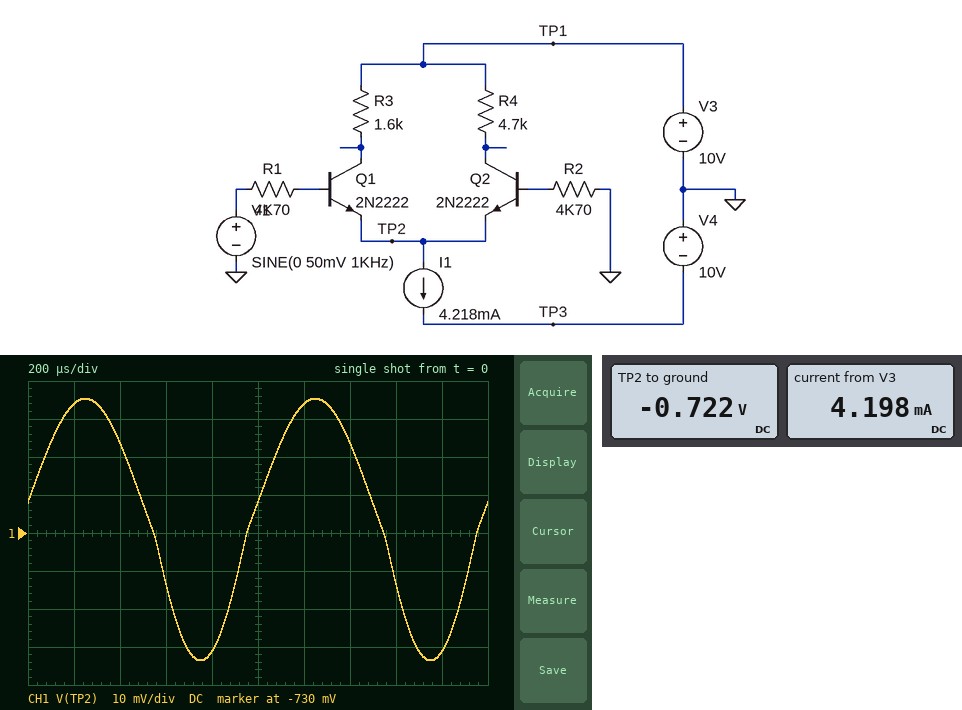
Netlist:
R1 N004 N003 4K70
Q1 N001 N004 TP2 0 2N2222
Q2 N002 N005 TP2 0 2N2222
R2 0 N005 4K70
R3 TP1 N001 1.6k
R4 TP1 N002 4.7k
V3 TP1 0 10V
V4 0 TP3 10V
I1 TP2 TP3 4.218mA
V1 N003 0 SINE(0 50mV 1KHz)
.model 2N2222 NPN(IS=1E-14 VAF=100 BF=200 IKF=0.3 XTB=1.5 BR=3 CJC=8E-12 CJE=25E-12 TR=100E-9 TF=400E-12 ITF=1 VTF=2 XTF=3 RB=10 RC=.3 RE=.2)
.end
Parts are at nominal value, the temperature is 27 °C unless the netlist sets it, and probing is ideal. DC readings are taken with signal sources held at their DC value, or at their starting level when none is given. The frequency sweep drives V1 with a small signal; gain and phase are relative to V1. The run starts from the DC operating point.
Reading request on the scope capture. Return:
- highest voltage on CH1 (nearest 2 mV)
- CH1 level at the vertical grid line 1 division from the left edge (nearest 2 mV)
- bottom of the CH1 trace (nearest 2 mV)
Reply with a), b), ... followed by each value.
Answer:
a) -694 mV
b) -696 mV
c) -764 mV
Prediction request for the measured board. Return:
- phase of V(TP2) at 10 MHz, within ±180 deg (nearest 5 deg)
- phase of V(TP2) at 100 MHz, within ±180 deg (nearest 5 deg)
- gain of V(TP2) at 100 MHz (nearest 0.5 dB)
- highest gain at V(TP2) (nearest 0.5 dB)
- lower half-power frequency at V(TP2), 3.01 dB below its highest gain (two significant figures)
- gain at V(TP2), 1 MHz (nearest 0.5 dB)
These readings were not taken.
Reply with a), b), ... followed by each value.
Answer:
a) -40 deg
b) -10 deg
c) -15.5 dB
d) -2.0 dB
e) 25 kHz
f) -2.0 dB
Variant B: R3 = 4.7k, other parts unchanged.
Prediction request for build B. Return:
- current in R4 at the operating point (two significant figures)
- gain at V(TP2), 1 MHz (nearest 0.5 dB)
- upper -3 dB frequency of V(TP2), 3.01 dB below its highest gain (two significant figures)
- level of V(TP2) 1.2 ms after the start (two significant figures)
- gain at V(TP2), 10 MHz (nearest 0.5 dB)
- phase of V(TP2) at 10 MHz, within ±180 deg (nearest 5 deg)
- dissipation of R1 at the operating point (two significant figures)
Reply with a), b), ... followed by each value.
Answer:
a) 2.1 mA
b) -6.5 dB
c) 3.2 MHz
d) -720 mV
e) -11.5 dB
f) -10 deg
g) 520 nW
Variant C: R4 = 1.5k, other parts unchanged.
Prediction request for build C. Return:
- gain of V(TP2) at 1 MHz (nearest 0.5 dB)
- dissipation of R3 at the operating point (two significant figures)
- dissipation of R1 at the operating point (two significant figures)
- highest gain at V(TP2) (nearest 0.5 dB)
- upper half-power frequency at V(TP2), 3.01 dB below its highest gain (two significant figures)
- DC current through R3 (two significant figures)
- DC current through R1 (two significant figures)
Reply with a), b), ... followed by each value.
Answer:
a) -6.5 dB
b) 7.0 mW
c) 460 nW
d) -6.0 dB
e) 6.8 MHz
f) 2.1 mA
g) 9.9 µA
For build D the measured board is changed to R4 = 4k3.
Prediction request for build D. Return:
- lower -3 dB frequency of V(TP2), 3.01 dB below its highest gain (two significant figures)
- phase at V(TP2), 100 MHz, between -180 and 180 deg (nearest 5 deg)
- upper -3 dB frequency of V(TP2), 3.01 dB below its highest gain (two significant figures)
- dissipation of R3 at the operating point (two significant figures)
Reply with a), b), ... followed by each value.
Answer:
a) 22 kHz
b) -10 deg
c) 5.7 MHz
d) 7.4 mW
